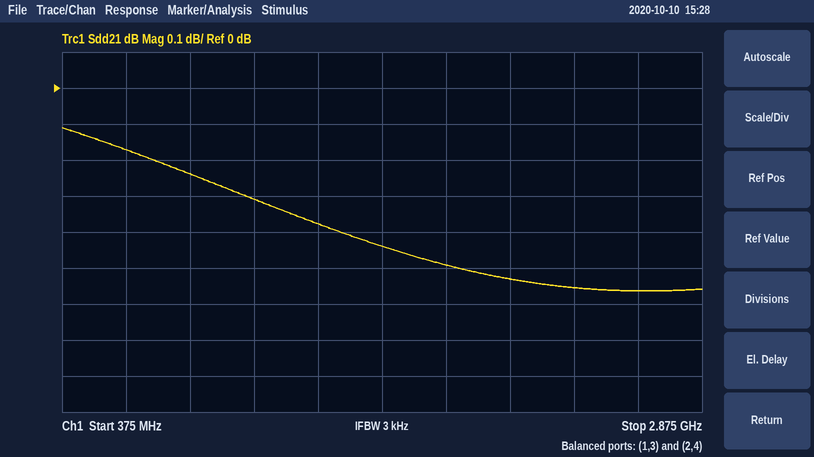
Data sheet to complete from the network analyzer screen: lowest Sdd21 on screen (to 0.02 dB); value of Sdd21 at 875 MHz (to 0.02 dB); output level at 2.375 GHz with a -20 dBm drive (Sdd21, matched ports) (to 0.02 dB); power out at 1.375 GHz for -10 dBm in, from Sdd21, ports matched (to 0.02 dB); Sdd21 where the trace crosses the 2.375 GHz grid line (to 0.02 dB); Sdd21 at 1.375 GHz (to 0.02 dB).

-0.56 dB
-0.24 dB
-20.56 dBm
-10.38 dBm
-0.56 dB
-0.38 dB
